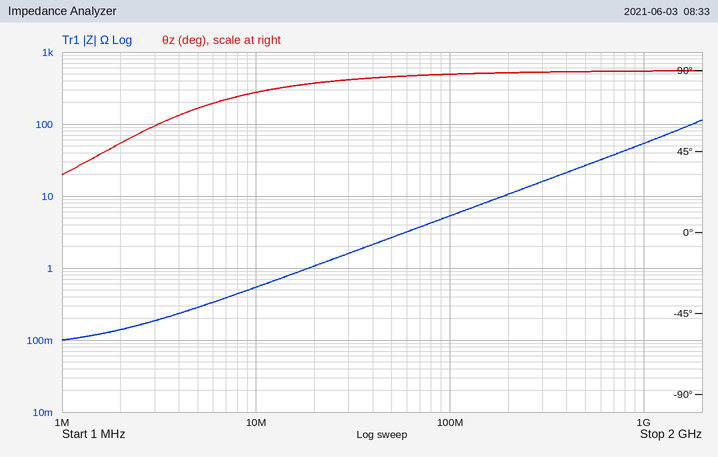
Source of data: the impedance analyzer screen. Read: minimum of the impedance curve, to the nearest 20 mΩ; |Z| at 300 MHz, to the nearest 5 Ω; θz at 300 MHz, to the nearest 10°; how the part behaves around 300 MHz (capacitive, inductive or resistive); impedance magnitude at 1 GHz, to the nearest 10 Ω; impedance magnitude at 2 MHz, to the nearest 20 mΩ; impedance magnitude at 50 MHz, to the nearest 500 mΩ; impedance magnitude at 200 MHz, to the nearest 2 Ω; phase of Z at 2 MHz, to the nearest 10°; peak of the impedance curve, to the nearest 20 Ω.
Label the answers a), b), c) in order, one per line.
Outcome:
a) 100 mΩ
b) 15 Ω
c) 90°
d) inductive
e) 50 Ω
f) 140 mΩ
g) 2.5 Ω
h) 10 Ω
i) 50°
j) 120 Ω
